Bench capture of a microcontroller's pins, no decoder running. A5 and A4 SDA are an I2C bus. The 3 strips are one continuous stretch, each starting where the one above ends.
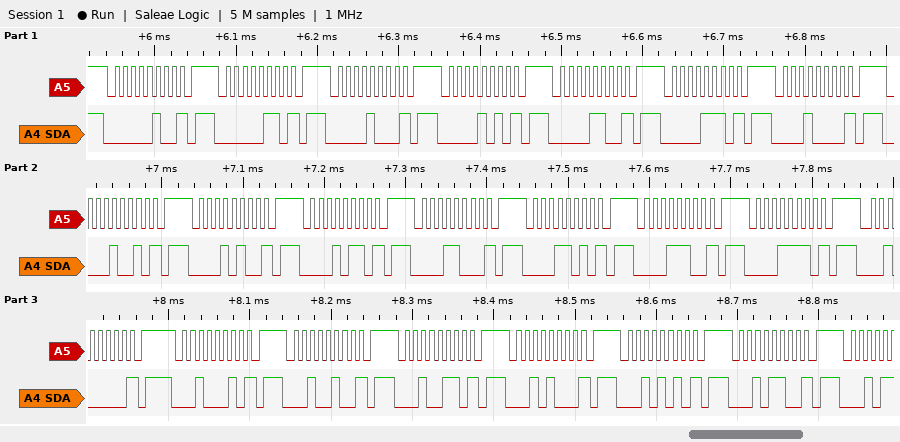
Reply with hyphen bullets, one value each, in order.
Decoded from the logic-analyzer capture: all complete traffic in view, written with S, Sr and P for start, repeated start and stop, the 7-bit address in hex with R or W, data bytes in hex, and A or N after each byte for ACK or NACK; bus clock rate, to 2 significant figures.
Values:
- S 02W N P S 03W N P S 04W N P S 05W N P S 06W N P S 07W N P S 08W N P S 09W N P S 0AW N P S 0BW N P S 0CW N P S 0DW N P S 0EW N P S 0FW N P S 10W N P S 11W N P S 12W N P S 13W N P S 14W N P S 15W N P S 16W N P
- 100 kHz
